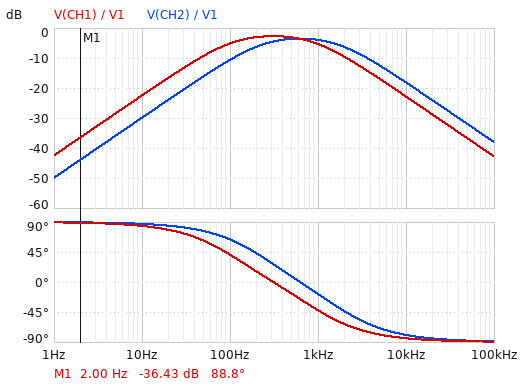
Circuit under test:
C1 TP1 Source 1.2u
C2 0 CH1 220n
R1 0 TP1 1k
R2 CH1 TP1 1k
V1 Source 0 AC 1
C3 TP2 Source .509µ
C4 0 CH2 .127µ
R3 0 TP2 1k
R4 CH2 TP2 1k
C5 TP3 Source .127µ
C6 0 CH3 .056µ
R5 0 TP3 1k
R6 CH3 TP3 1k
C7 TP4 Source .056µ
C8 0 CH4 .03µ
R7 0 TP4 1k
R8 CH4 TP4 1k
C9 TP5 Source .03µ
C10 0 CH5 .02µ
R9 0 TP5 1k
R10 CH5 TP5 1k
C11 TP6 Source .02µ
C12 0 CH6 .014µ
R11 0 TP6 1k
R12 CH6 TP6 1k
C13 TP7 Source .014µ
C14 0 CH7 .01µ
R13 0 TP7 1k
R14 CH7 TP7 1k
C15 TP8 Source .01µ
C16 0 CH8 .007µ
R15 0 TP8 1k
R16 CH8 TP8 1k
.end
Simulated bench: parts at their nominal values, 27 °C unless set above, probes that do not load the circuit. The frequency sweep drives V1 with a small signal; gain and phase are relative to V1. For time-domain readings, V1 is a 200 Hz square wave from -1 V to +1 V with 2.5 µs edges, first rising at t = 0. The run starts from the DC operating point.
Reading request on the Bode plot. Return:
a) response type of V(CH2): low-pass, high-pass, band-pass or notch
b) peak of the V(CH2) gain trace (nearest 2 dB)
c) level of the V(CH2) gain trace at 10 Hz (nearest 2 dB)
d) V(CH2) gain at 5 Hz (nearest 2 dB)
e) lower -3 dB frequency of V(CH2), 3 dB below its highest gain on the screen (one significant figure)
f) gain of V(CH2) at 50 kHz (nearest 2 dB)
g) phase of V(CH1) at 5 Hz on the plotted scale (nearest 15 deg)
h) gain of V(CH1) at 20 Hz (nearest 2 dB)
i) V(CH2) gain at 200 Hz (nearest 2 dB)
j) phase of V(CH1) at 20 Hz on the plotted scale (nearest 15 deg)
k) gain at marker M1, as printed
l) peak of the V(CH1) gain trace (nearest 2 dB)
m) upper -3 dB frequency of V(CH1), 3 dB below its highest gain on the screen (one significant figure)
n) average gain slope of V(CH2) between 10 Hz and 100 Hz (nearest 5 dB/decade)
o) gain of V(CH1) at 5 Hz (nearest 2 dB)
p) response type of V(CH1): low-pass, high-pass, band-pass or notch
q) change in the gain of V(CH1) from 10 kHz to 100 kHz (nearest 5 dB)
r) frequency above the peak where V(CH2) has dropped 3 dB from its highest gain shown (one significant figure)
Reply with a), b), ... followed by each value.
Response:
a) band-pass
b) -4 dB
c) -30 dB
d) -36 dB
e) 200 Hz
f) -32 dB
g) 90 deg
h) -16 dB
i) -6 dB
j) 75 deg
k) -36.43 dB
l) -2 dB
m) 1 kHz
n) 20 dB/decade
o) -28 dB
p) band-pass
q) -20 dB
r) 2 kHz
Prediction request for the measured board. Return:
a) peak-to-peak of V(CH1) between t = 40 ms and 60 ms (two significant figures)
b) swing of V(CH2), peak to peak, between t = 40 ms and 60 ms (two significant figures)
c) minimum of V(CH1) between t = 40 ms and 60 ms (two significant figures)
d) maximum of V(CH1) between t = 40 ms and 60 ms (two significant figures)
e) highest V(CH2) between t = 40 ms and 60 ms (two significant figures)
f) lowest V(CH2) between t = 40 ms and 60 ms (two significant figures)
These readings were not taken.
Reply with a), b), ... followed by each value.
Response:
a) 2.0 V
b) 2.1 V
c) -1.0 V
d) 1.0 V
e) 1.1 V
f) -1.1 V
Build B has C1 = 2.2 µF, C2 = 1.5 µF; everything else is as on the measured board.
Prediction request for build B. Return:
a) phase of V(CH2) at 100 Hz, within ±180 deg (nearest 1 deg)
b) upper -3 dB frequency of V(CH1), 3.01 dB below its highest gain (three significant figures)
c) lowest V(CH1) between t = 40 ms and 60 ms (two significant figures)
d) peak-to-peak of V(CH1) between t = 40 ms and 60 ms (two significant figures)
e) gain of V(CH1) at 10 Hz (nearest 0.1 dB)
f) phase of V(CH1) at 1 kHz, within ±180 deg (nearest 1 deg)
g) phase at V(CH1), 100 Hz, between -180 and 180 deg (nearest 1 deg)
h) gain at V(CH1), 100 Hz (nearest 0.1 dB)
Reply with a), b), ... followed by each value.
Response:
a) 64 deg
b) 278 Hz
c) -400 mV
d) 810 mV
e) -17.5 dB
f) -76 deg
g) -5 deg
h) -7.5 dB
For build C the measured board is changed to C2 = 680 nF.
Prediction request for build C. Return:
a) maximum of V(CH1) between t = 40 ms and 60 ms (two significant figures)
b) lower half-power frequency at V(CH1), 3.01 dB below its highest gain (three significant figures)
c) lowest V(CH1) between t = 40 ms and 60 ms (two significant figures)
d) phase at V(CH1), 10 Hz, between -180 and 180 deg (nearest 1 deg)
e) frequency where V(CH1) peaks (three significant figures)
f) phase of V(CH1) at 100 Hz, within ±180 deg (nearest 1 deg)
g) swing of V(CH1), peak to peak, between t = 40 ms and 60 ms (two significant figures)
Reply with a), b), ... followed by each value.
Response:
a) 550 mV
b) 55.9 Hz
c) -550 mV
d) 81 deg
e) 176 Hz
f) 23 deg
g) 1.1 V
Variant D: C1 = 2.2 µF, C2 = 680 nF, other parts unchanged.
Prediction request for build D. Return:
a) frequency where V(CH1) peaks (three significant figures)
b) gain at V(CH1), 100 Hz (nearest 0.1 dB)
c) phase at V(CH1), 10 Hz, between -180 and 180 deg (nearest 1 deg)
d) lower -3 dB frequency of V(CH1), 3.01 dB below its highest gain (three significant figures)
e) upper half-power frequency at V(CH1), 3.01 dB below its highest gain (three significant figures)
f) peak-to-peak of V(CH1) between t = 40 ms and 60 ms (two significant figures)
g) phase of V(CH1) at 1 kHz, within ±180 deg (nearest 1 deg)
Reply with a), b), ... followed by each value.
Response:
a) 130 Hz
b) -4.3 dB
c) 77 deg
d) 40.4 Hz
e) 419 Hz
f) 1.3 V
g) -69 deg
